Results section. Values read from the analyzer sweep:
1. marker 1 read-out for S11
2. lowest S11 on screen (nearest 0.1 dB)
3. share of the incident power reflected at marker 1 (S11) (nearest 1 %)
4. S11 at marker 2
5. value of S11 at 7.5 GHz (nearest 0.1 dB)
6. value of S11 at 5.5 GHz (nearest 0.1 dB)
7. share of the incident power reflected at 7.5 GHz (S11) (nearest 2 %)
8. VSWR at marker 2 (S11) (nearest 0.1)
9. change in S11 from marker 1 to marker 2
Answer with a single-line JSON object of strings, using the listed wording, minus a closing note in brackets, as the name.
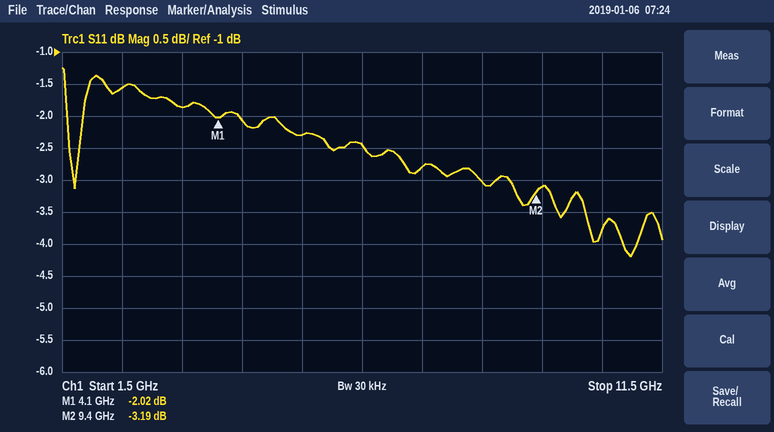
{"marker 1 read-out for S11": "-2.02 dB", "lowest S11 on screen": "-4.2 dB", "share of the incident power reflected at marker 1 (S11)": "63 %", "S11 at marker 2": "-3.19 dB", "value of S11 at 7.5 GHz": "-2.8 dB", "value of S11 at 5.5 GHz": "-2.3 dB", "share of the incident power reflected at 7.5 GHz (S11)": "52 %", "VSWR at marker 2 (S11)": "5.5", "change in S11 from marker 1 to marker 2": "-1.17 dB"}
